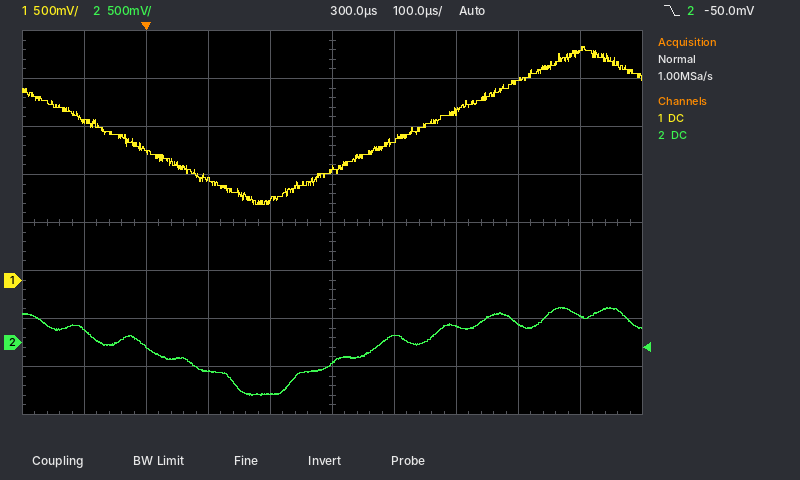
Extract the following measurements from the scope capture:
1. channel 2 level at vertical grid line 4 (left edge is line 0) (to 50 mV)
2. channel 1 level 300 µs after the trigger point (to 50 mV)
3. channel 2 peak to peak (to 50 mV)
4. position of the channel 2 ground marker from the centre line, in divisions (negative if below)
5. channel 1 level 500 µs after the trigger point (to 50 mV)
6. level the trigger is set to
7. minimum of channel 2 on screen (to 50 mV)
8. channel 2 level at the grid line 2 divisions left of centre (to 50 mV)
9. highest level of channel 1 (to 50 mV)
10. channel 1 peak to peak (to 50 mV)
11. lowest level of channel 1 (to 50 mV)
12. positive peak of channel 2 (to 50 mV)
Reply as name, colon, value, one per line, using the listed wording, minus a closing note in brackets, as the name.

channel 2 level at vertical grid line 4 (left edge is line 0): -550 mV
channel 1 level 300 µs after the trigger point: 1.15 V
channel 2 peak to peak: 900 mV
position of the channel 2 ground marker from the centre line, in divisions: -2.5 div
channel 1 level 500 µs after the trigger point: 1.75 V
level the trigger is set to: -50.0 mV
minimum of channel 2 on screen: -550 mV
channel 2 level at the grid line 2 divisions left of centre: -300 mV
highest level of channel 1: 2.45 V
channel 1 peak to peak: 1.65 V
lowest level of channel 1: 800 mV
positive peak of channel 2: 350 mV
